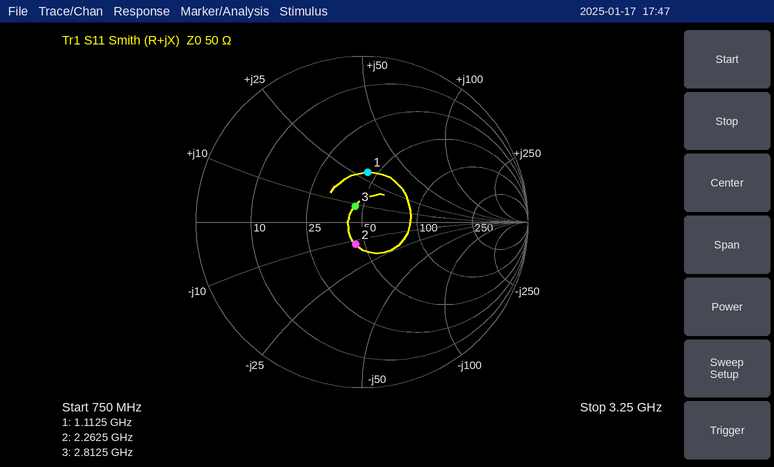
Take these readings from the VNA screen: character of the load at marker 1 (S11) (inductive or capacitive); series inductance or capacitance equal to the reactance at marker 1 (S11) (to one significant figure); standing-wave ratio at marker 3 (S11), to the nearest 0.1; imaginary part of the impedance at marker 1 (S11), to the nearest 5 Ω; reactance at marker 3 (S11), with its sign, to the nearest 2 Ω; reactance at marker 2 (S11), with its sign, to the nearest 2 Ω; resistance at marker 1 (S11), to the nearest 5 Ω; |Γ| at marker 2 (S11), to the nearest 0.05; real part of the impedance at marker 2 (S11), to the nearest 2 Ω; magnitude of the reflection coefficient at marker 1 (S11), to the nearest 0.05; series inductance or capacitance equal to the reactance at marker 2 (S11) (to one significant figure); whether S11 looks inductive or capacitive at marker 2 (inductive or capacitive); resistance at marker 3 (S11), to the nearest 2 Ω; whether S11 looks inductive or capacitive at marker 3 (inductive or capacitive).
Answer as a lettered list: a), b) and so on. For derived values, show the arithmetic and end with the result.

a) inductive
b) L = 30 Ω/(2π × 1.1125 GHz) ≈ 4 nH
c) 1.2
d) +30 Ω
e) +8 Ω
f) -12 Ω
g) 45 Ω
h) 0.15
i) 44 Ω
j) 0.30
k) C = 1/(2π × 2.2625 GHz × 12 Ω) ≈ 6 pF
l) capacitive
m) 46 Ω
n) inductive
